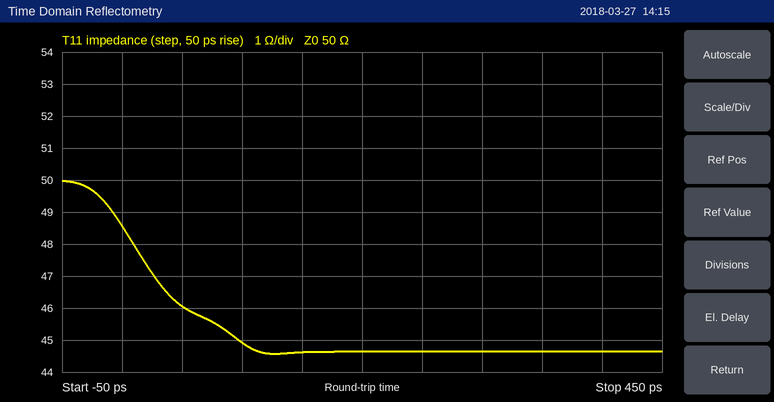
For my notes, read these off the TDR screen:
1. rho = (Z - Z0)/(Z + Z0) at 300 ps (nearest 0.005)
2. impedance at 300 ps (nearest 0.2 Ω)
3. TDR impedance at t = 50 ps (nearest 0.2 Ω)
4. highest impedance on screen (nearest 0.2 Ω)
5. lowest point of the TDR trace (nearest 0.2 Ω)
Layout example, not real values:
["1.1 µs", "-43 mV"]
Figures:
["-0.055", "44.6 Ω", "46.0 Ω", "50.0 Ω", "44.6 Ω"]
